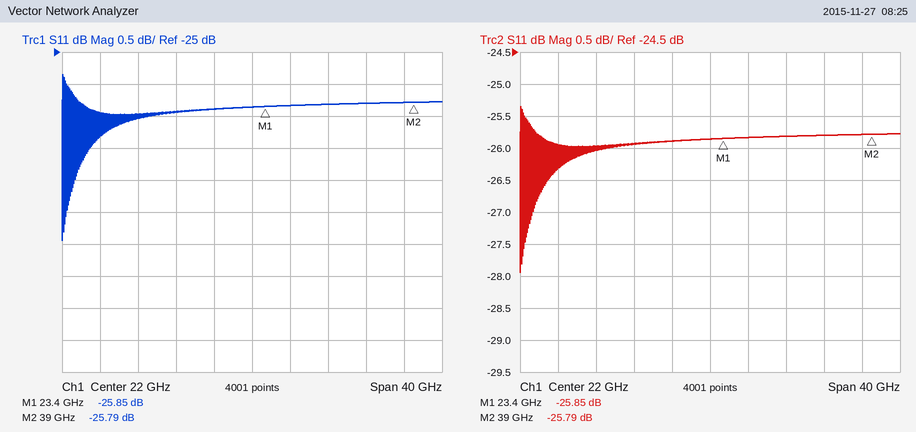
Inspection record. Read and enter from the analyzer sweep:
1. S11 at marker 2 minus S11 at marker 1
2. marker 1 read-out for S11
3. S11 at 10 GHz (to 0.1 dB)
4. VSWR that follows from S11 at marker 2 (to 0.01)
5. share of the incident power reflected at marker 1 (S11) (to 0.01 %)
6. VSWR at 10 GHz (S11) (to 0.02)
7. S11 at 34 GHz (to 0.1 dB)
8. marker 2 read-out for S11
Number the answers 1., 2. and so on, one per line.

1. 0.06 dB
2. -25.85 dB
3. -26.0 dB
4. 1.11
5. 0.26 %
6. 1.10
7. -25.8 dB
8. -25.79 dB
